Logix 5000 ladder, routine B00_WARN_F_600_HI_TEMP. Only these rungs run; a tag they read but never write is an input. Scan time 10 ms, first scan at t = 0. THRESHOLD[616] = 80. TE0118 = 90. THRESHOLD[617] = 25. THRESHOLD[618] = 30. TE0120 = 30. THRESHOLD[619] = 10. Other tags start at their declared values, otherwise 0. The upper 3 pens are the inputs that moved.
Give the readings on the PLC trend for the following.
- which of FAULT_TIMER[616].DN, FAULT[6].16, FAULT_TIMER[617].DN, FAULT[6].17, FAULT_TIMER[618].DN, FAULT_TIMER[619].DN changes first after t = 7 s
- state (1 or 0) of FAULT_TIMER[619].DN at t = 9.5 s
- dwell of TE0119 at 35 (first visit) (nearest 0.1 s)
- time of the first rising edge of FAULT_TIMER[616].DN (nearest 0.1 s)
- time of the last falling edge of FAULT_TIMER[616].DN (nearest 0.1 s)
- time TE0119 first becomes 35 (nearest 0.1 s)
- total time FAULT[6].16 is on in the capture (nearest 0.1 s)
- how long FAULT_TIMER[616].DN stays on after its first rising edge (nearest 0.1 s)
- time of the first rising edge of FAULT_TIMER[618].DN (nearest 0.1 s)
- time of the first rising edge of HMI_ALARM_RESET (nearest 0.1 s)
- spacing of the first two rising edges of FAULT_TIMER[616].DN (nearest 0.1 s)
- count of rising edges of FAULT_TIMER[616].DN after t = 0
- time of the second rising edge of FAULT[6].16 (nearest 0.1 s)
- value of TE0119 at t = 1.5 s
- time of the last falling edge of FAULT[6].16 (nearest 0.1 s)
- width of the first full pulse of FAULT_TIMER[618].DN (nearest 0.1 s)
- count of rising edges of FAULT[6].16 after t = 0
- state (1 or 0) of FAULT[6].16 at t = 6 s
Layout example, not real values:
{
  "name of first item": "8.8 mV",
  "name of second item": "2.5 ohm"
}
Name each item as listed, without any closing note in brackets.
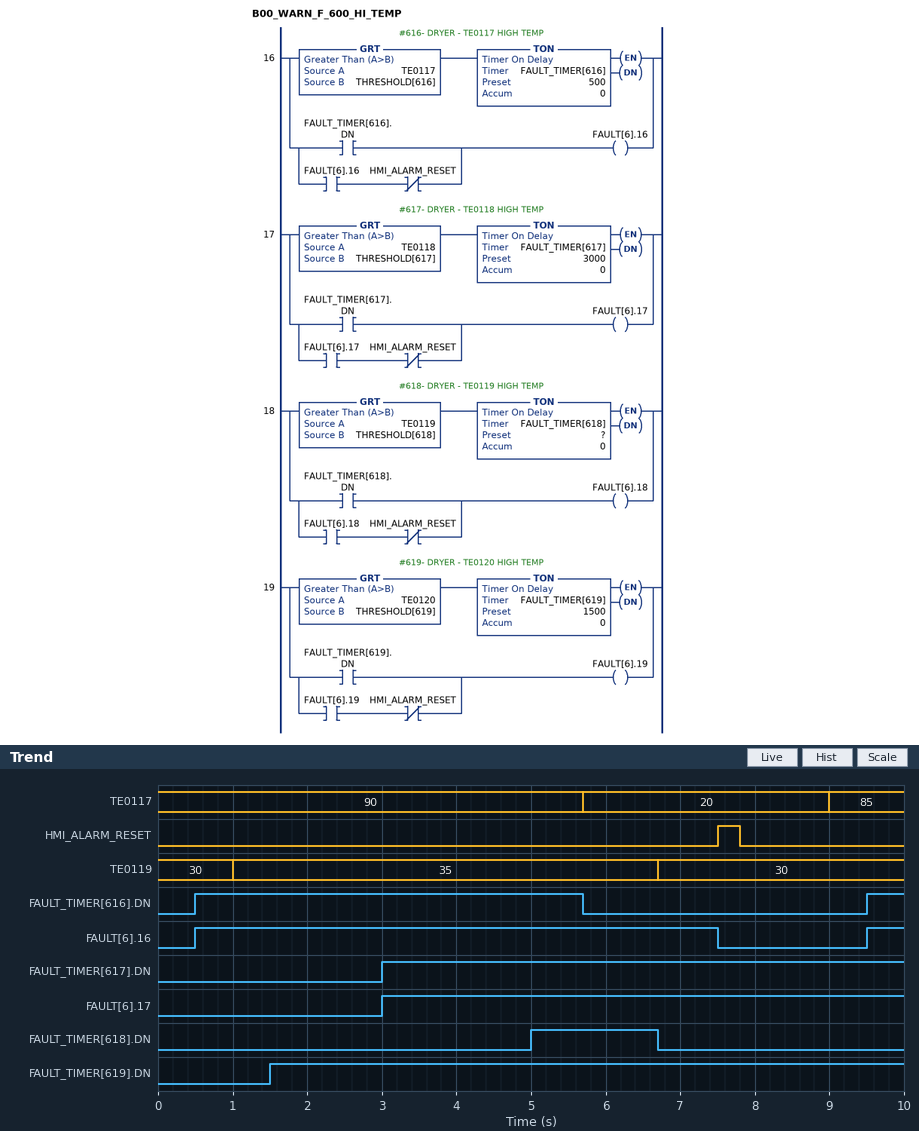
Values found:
{
  "which of FAULT_TIMER[616].DN, FAULT[6].16, FAULT_TIMER[617].DN, FAULT[6].17, FAULT_TIMER[618].DN, FAULT_TIMER[619].DN changes first after t = 7 s": "FAULT[6].16",
  "state (1 or 0) of FAULT_TIMER[619].DN at t = 9.5 s": "1",
  "dwell of TE0119 at 35 (first visit)": "5.7 s",
  "time of the first rising edge of FAULT_TIMER[616].DN": "0.5 s",
  "time of the last falling edge of FAULT_TIMER[616].DN": "5.7 s",
  "time TE0119 first becomes 35": "1.0 s",
  "total time FAULT[6].16 is on in the capture": "7.5 s",
  "how long FAULT_TIMER[616].DN stays on after its first rising edge": "5.2 s",
  "time of the first rising edge of FAULT_TIMER[618].DN": "5.0 s",
  "time of the first rising edge of HMI_ALARM_RESET": "7.5 s",
  "spacing of the first two rising edges of FAULT_TIMER[616].DN": "9.0 s",
  "count of rising edges of FAULT_TIMER[616].DN after t = 0": "2",
  "time of the second rising edge of FAULT[6].16": "9.5 s",
  "value of TE0119 at t = 1.5 s": "35",
  "time of the last falling edge of FAULT[6].16": "7.5 s",
  "width of the first full pulse of FAULT_TIMER[618].DN": "1.7 s",
  "count of rising edges of FAULT[6].16 after t = 0": "2",
  "state (1 or 0) of FAULT[6].16 at t = 6 s": "1"
}
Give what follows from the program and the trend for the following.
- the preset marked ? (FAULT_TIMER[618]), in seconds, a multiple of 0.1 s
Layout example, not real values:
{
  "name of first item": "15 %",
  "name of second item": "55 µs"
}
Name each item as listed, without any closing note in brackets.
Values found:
{
  "the preset marked ? (FAULT_TIMER[618]), in seconds, a multiple of 0.1 s": "4.0 s"
}
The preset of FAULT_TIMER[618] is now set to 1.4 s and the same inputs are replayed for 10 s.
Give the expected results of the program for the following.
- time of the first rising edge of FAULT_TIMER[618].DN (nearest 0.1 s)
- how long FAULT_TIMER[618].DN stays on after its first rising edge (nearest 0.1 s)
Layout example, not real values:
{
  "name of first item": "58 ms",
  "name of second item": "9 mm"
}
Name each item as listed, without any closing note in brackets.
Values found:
{
  "time of the first rising edge of FAULT_TIMER[618].DN": "2.4 s",
  "how long FAULT_TIMER[618].DN stays on after its first rising edge": "4.3 s"
}
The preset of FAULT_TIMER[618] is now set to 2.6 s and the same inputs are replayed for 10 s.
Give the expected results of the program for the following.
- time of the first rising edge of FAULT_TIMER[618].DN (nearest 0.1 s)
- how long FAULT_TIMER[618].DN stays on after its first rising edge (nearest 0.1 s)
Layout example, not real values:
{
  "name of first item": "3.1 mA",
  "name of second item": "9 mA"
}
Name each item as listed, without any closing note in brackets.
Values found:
{
  "time of the first rising edge of FAULT_TIMER[618].DN": "3.6 s",
  "how long FAULT_TIMER[618].DN stays on after its first rising edge": "3.1 s"
}
